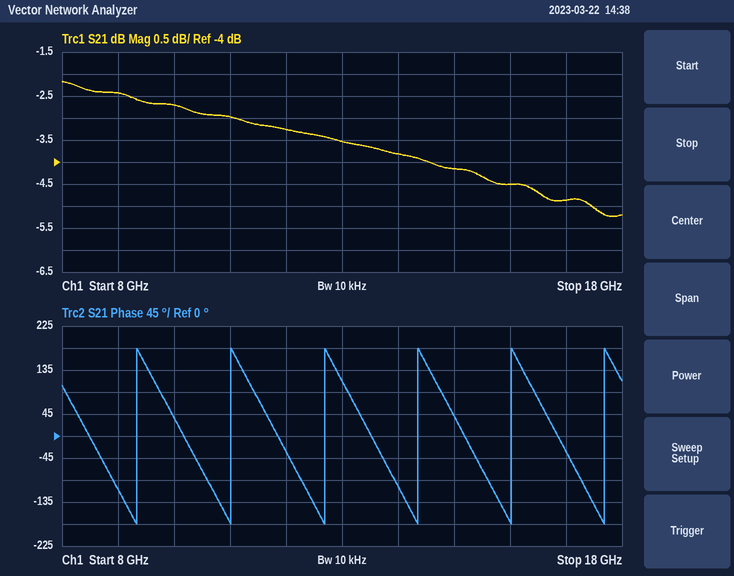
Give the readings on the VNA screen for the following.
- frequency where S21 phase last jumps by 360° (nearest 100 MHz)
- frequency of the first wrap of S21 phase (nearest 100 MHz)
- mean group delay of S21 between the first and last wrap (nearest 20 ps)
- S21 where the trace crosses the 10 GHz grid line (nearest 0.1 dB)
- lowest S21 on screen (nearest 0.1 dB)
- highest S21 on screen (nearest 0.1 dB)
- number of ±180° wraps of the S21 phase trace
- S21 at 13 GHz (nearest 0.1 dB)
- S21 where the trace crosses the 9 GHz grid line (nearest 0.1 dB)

17.7 GHz
9.3 GHz
600 ps
-2.7 dB
-5.2 dB
-2.2 dB
6
-3.5 dB
-2.4 dB
